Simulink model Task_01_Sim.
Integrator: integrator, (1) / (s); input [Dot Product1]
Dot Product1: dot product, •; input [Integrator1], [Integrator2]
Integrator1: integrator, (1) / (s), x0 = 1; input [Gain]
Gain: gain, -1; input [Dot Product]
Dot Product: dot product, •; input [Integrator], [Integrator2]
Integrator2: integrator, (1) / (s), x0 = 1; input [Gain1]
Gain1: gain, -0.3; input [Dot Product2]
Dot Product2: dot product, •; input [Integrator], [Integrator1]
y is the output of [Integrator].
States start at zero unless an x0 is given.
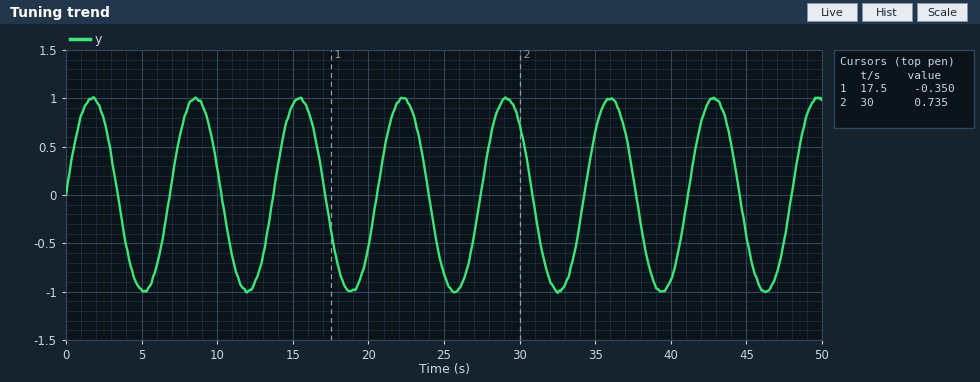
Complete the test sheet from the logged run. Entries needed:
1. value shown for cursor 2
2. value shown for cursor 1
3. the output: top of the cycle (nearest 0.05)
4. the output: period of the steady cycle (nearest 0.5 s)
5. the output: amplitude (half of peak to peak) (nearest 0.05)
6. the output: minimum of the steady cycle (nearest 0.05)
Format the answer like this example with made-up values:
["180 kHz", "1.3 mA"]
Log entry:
["0.735", "-0.350", "1.00", "7.0 s", "1.00", "-1.00"]
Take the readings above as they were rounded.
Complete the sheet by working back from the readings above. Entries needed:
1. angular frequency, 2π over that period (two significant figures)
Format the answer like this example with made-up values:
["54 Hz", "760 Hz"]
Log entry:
["0.90 rad/s"]
